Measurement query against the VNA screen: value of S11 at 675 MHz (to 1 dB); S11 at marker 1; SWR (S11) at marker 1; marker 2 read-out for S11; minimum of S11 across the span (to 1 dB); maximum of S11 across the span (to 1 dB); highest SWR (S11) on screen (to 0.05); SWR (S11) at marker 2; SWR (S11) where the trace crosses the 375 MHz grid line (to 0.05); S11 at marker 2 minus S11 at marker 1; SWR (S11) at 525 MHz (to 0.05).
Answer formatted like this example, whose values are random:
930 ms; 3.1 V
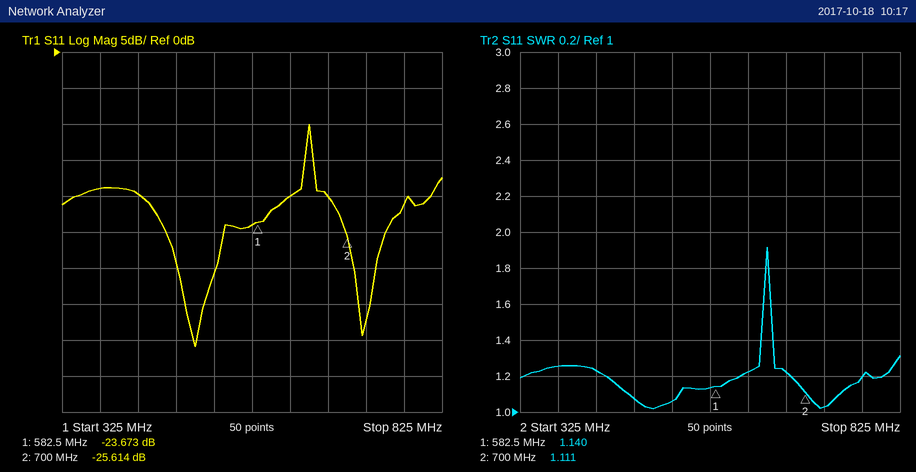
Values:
-20 dB; -23.673 dB; 1.140; -25.614 dB; -41 dB; -10 dB; 1.90; 1.111; 1.25; -1.941 dB; 1.05
